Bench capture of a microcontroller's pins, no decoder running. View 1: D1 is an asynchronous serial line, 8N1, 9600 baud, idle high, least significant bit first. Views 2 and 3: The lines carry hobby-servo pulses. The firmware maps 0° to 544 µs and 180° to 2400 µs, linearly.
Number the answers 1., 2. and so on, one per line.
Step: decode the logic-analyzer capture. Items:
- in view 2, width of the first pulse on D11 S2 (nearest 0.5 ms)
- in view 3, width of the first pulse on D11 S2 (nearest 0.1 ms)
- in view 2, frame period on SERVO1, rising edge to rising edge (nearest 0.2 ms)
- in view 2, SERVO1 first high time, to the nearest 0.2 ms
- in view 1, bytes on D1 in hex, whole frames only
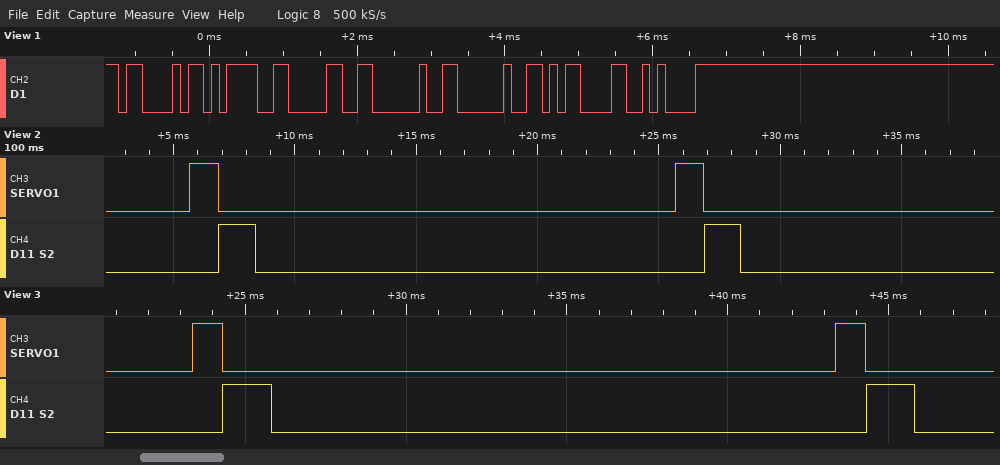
1. 1.5 ms
2. 1.5 ms
3. 20.0 ms
4. 1.2 ms
5. 0x43 0x3D 0x30 0x20 0x20 0x0D 0x0A
